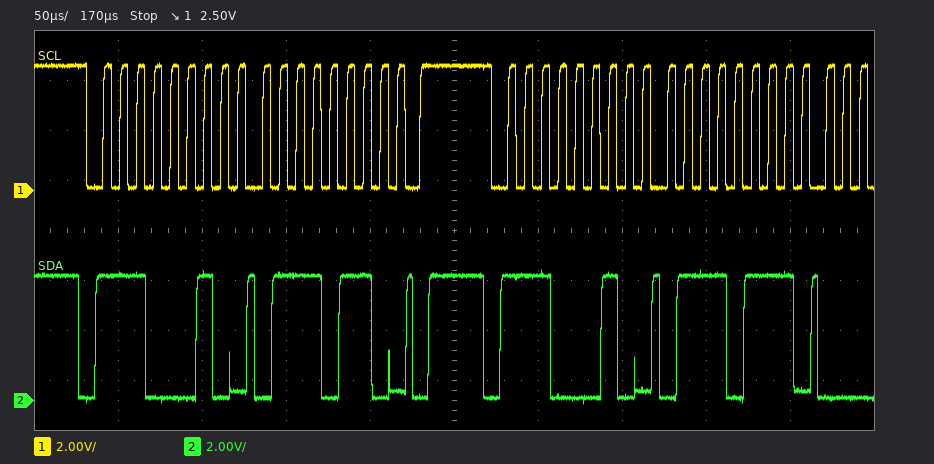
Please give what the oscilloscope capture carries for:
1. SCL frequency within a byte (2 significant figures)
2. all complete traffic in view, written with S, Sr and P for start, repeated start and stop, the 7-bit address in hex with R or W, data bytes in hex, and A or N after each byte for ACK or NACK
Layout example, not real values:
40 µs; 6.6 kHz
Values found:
100 kHz; S 71W A 76 A P S 71W A 77 A
